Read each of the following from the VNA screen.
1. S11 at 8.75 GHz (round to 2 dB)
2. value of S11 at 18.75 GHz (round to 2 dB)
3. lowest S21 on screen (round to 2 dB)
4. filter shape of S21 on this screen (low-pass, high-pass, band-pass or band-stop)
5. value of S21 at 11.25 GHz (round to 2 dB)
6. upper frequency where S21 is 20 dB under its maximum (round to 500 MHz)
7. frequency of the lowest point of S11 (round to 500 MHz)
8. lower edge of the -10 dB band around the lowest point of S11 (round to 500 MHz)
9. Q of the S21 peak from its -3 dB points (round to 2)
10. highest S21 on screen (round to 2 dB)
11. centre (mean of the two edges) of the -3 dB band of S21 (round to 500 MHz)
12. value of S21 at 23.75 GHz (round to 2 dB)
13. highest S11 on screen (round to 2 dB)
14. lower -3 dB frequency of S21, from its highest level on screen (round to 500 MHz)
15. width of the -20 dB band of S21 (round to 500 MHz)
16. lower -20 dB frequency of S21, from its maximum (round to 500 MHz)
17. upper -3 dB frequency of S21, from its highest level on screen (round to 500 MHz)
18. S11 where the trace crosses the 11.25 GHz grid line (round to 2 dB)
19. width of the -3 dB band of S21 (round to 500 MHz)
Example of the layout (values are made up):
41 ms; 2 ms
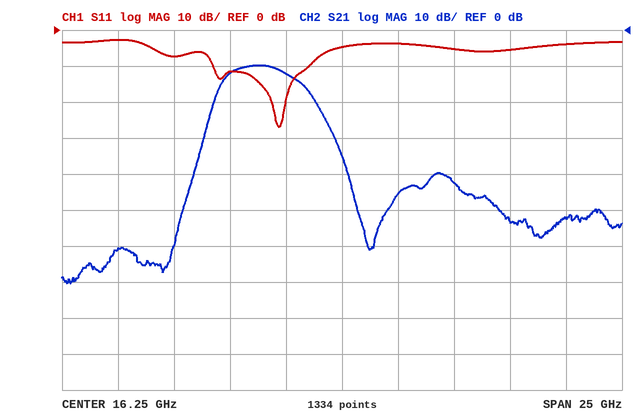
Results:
-8 dB; -4 dB; -70 dB; band-pass; -12 dB; 16.0 GHz; 13.5 GHz; 10.5 GHz; 4; -10 dB; 12.5 GHz; -54 dB; -2 dB; 11.0 GHz; 6.0 GHz; 10.0 GHz; 14.0 GHz; -12 dB; 3.0 GHz
